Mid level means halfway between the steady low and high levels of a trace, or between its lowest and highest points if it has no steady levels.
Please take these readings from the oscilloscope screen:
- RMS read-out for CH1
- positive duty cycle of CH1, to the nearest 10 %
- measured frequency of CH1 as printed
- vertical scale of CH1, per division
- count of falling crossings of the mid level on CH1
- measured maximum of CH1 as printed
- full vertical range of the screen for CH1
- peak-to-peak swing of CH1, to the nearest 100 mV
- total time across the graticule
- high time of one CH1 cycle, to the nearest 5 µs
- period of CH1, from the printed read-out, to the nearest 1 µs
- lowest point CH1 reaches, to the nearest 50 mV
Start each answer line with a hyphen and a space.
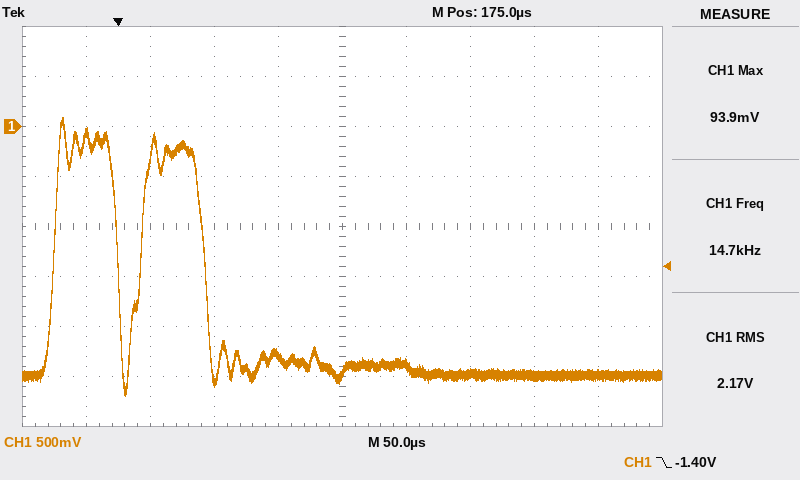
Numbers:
- 2.17 V
- 70 %
- 14.7 kHz
- 500 mV
- 2
- 93.9 mV
- 4 V
- 2.80 V
- 500 µs
- 50 µs
- 68 µs
- -2.70 V
